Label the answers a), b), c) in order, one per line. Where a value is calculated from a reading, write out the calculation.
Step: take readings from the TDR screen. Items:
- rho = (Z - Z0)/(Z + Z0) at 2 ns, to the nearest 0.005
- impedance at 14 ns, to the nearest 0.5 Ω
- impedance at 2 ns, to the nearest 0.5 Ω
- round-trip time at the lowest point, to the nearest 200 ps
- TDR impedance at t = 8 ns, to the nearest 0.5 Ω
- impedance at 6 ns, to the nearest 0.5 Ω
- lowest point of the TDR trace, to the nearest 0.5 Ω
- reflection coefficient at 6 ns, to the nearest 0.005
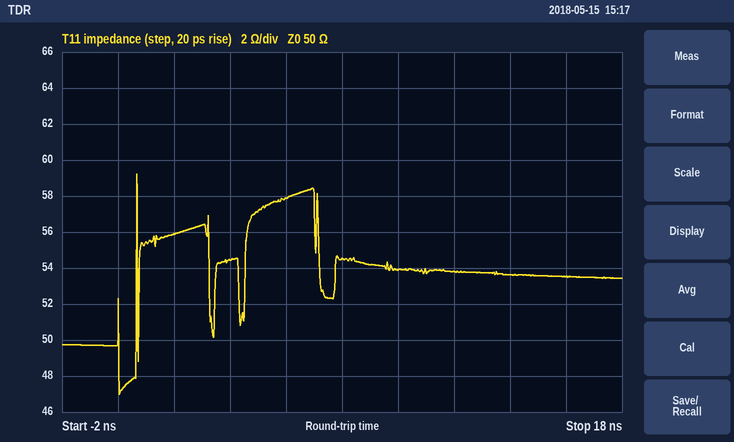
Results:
a) (56 − 50)/(56 + 50) ≈ +0.0566, so +0.055 to the nearest 0.005
b) 53.5 Ω
c) 56.0 Ω
d) 0.0 ns
e) 54.5 Ω
f) 58.0 Ω
g) 47.0 Ω
h) (58 − 50)/(58 + 50) ≈ +0.0741, so +0.075 to the nearest 0.005
